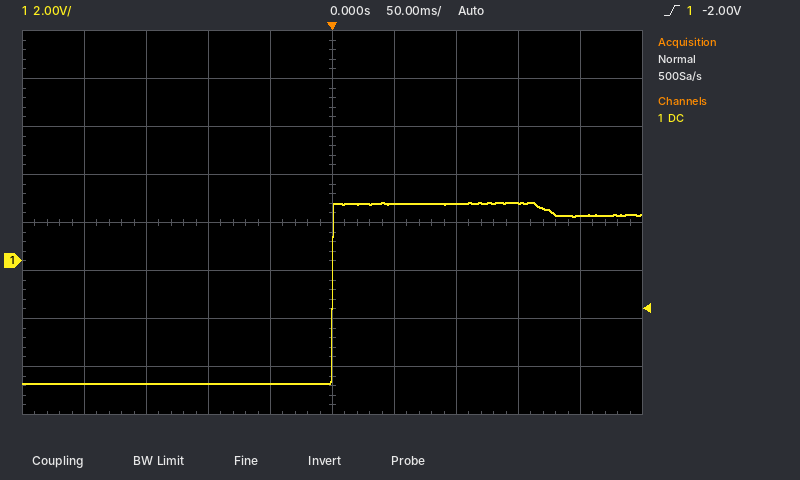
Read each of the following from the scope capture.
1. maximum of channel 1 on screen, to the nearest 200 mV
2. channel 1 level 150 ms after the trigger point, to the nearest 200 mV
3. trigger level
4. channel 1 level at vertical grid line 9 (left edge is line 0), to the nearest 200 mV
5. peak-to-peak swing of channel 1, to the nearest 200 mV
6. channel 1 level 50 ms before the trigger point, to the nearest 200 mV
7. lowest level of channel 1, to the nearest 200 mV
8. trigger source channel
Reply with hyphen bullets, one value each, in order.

- 2.4 V
- 2.4 V
- -2.00 V
- 1.8 V
- 7.6 V
- -5.2 V
- -5.2 V
- channel 1
